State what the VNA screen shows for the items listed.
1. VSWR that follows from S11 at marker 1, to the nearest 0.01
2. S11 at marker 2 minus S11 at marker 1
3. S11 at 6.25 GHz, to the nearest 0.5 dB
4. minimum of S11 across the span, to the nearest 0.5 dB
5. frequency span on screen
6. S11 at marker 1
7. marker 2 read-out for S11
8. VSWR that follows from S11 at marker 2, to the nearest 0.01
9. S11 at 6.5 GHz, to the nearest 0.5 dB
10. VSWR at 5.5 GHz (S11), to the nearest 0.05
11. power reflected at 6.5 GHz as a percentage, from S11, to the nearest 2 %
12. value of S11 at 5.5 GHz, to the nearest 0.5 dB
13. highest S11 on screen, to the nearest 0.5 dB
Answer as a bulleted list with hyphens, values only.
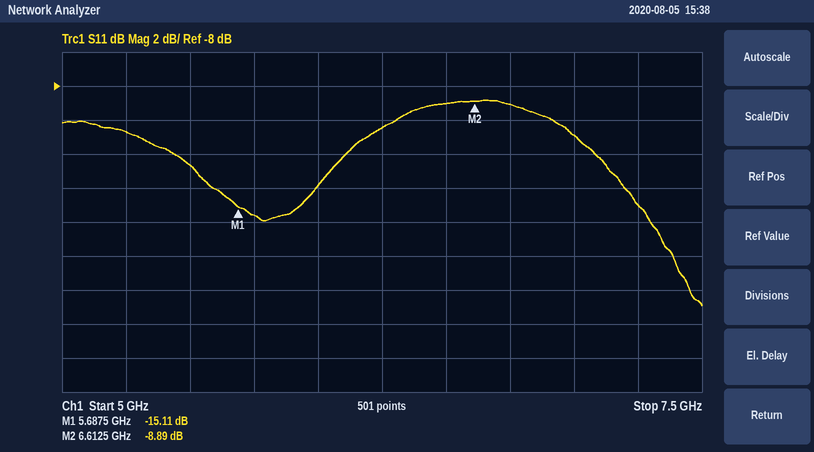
- 1.43
- 6.22 dB
- -10.5 dB
- -21.0 dB
- 2.5 GHz
- -15.11 dB
- -8.89 dB
- 2.12
- -9.0 dB
- 1.60
- 12 %
- -12.5 dB
- -9.0 dB
